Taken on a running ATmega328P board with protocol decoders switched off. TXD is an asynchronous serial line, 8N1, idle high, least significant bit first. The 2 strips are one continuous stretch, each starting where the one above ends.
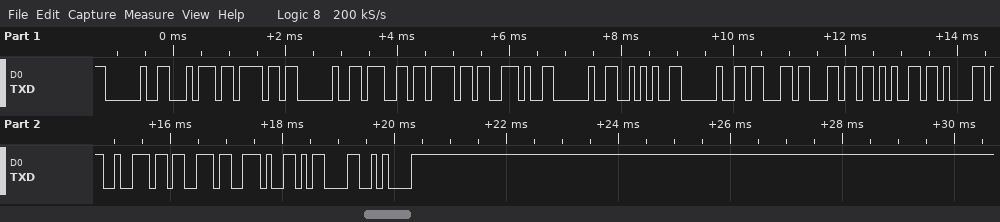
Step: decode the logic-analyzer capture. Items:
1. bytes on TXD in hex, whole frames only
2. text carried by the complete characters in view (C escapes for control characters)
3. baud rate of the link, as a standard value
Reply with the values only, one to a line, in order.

20 74 6F 20 67 6F 2E 20 2A 20 63 6C 65 61 72 73 2E 0D 0A
" to go. * clears.\r\n"
9600 baud
